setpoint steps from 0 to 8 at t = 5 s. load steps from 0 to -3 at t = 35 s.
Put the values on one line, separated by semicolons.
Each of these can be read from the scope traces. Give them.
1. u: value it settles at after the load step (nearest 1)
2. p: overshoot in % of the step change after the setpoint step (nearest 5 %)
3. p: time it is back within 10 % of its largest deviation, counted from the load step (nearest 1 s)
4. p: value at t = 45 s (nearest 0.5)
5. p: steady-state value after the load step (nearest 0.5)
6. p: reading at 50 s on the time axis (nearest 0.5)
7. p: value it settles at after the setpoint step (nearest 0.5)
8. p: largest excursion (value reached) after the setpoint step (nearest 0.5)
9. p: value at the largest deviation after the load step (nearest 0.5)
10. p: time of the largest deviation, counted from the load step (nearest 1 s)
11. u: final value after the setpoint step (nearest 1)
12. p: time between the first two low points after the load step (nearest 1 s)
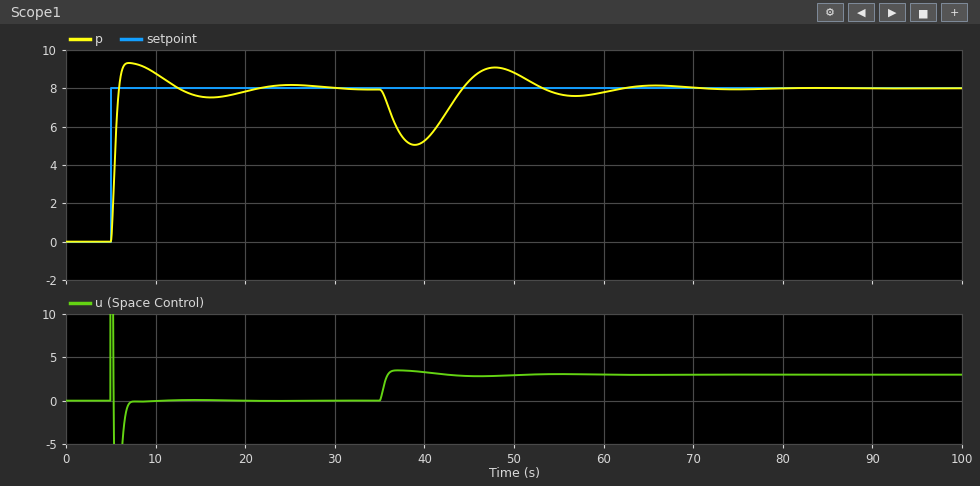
3; 15 %; 24 s; 8.5; 8.0; 9.0; 8.0; 9.5; 5.0; 4 s; 0; 18 s
